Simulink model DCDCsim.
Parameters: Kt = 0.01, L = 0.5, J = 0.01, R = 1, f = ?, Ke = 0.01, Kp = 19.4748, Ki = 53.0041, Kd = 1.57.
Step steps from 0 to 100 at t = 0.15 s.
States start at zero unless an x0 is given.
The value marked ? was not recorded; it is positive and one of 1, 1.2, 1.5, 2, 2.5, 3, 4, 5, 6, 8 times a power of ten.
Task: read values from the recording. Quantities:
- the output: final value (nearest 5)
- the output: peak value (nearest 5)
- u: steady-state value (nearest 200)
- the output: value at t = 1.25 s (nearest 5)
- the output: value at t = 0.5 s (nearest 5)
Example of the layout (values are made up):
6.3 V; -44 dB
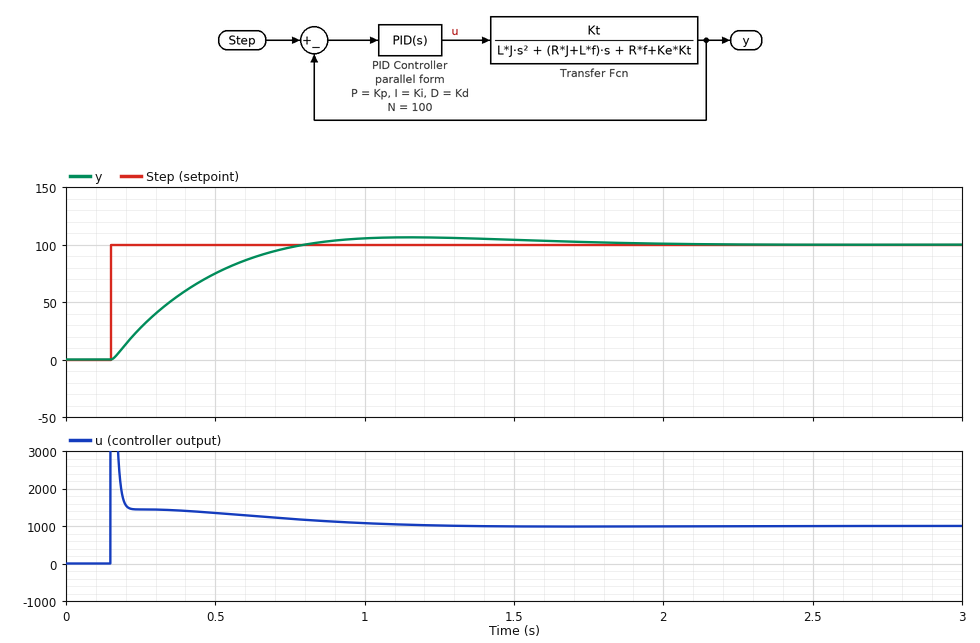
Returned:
100; 105; 1000; 105; 75
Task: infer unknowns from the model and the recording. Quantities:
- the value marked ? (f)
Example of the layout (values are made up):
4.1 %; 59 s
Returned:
0.1
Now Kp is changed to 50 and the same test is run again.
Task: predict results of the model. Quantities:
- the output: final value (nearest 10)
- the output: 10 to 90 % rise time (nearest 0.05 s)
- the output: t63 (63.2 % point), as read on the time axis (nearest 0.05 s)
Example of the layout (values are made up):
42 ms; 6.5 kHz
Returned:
100; 0.20 s; 0.30 s
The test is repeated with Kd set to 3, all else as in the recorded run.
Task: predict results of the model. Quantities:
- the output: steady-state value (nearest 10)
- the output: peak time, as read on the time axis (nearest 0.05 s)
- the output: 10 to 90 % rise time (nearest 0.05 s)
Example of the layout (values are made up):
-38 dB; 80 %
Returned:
100; 1.35 s; 0.55 s
